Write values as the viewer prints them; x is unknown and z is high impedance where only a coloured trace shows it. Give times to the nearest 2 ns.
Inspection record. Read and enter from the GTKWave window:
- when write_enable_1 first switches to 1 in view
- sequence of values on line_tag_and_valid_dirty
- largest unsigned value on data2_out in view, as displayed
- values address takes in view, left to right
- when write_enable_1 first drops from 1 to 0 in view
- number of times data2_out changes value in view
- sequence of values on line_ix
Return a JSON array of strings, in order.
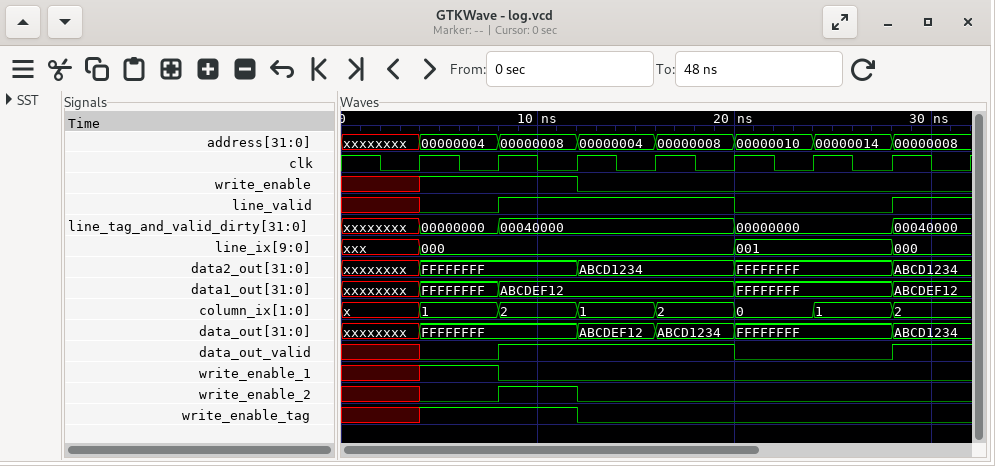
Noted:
["4 ns", "xxxxxxxx, 00000000, 00040000, 00000000, 00040000", "FFFFFFFF", "xxxxxxxx, 00000004, 00000008, 00000004, 00000008, 00000010, 00000014, 00000008", "8 ns", "4", "xxx, 000, 001, 000"]
